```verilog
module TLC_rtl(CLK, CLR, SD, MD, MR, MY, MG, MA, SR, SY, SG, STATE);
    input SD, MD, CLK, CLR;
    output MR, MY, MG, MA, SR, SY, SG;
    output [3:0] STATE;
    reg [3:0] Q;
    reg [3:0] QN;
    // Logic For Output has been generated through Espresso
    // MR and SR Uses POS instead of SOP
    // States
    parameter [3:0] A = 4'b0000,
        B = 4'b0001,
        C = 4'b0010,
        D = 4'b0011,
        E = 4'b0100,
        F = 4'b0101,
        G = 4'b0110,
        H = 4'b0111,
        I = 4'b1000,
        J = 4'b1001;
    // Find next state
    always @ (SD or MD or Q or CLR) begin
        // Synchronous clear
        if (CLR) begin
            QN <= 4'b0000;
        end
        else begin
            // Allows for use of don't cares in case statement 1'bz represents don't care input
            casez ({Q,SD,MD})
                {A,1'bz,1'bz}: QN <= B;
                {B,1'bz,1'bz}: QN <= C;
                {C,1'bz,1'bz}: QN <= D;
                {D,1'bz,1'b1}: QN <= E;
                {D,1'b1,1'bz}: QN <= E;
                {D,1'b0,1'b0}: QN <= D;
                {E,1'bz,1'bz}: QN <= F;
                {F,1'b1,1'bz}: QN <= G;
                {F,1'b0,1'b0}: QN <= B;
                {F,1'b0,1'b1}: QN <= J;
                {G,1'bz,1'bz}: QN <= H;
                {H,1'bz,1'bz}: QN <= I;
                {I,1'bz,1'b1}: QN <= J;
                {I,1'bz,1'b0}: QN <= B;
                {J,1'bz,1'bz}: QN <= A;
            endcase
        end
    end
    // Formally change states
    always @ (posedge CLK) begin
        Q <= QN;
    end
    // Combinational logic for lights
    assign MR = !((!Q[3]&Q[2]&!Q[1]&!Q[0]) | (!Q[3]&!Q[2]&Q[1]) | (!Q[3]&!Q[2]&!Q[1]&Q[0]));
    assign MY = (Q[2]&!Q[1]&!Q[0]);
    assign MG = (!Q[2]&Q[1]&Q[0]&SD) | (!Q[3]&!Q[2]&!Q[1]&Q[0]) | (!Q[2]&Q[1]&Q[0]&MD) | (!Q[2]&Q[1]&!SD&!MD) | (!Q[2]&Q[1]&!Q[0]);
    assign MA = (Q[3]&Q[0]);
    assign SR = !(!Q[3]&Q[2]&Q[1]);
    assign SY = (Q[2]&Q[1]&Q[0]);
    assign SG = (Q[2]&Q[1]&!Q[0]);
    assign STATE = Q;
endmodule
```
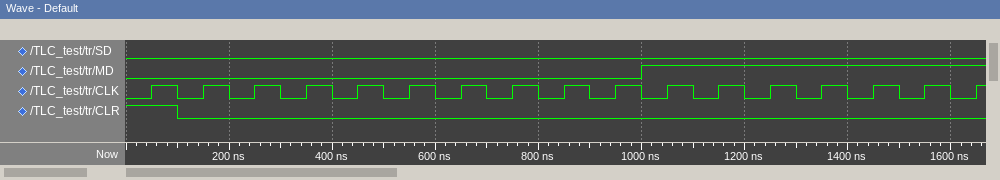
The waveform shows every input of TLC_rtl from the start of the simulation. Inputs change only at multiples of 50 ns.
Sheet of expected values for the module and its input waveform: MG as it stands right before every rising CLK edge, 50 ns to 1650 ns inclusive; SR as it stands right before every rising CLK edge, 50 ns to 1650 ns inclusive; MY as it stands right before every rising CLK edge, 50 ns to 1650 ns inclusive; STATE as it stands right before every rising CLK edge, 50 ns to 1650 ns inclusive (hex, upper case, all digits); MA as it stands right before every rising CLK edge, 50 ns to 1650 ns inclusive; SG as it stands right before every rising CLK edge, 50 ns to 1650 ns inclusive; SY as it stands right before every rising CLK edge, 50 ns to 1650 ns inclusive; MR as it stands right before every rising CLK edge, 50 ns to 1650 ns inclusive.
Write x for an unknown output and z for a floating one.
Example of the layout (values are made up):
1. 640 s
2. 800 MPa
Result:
1. x 0 1 1 1 1 1 1 1 1 1 0 0 0 0 1 1
2. x 1 1 1 1 1 1 1 1 1 1 1 1 1 1 1 1
3. x 0 0 0 0 0 0 0 0 0 0 1 0 0 0 0 0
4. x, 0, 1, 2, 3, 3, 3, 3, 3, 3, 3, 4, 5, 9, 0, 1, 2
5. x 0 0 0 0 0 0 0 0 0 0 0 0 1 0 0 0
6. x 0 0 0 0 0 0 0 0 0 0 0 0 0 0 0 0
7. x 0 0 0 0 0 0 0 0 0 0 0 0 0 0 0 0
8. x 1 0 0 0 0 0 0 0 0 0 0 1 1 1 0 0
